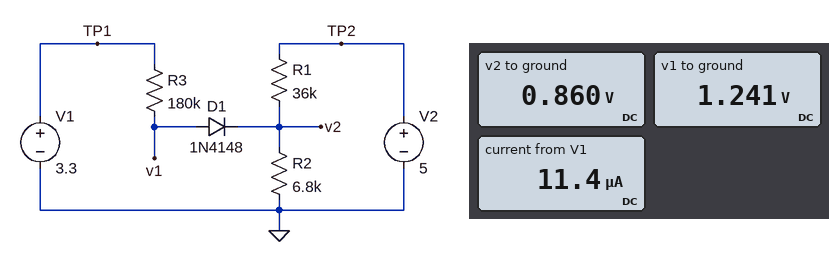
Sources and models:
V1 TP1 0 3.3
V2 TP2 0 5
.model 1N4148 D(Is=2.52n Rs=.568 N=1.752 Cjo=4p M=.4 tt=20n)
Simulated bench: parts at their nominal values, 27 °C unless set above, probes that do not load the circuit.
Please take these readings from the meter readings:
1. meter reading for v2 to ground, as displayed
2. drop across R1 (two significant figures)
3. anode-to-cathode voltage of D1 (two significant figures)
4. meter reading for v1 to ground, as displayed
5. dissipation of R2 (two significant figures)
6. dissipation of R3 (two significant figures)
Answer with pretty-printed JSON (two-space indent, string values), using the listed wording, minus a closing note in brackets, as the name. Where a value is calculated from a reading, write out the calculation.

{
  "meter reading for v2 to ground, as displayed": "0.860 V",
  "drop across R1": "5 V - 860 mV = 4.1 V",
  "anode-to-cathode voltage of D1": "1.241 V - 860 mV = 380 mV",
  "meter reading for v1 to ground, as displayed": "1.241 V",
  "dissipation of R2": "(860 mV)^2 / 6.8 kΩ = 110 µW",
  "dissipation of R3": "(3.3 V - 1.241 V)^2 / 180 kΩ = 24 µW"
}
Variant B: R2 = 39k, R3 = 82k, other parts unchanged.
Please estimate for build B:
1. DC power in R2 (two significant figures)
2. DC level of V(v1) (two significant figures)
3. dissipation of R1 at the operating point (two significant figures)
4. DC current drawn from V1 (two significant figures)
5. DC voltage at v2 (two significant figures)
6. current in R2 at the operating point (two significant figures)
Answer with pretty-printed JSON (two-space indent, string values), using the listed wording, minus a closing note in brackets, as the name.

{
  "DC power in R2": "180 µW",
  "DC level of V(v1)": "3.0 V",
  "dissipation of R1 at the operating point": "150 µW",
  "DC current drawn from V1": "3.7 µA",
  "DC voltage at v2": "2.7 V",
  "current in R2 at the operating point": "68 µA"
}
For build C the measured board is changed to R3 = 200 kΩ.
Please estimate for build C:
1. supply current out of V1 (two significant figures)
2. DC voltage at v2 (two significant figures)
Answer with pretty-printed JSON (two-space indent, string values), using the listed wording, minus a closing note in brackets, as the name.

{
  "supply current out of V1": "10 µA",
  "DC voltage at v2": "850 mV"
}
